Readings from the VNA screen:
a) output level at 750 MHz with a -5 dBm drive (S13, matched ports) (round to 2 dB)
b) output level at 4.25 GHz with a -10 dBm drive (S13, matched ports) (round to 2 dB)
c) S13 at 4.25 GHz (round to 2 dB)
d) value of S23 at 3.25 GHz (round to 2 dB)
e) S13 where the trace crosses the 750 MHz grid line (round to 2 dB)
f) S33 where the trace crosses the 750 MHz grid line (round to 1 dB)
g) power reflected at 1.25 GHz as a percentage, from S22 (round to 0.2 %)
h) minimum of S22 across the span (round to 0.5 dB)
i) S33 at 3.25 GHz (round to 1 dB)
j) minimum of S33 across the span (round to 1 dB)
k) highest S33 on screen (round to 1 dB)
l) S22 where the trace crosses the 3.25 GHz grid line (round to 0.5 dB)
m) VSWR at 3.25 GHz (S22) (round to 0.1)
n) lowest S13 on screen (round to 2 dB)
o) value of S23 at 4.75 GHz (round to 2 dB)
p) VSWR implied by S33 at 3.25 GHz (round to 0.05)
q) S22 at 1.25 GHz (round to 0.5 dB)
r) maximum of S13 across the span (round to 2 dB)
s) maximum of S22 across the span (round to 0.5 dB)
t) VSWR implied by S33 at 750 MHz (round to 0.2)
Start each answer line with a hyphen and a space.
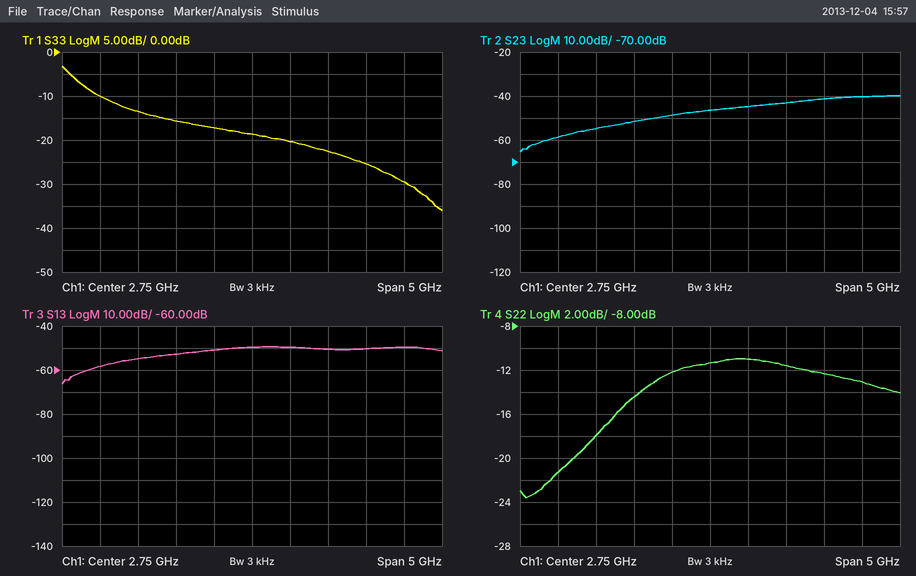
- -64 dBm
- -60 dBm
- -50 dB
- -44 dB
- -58 dB
- -10 dB
- 1.6 %
- -23.5 dB
- -20 dB
- -36 dB
- -3 dB
- -11.0 dB
- 1.8
- -66 dB
- -40 dB
- 1.20
- -18.0 dB
- -50 dB
- -11.0 dB
- 2.0
